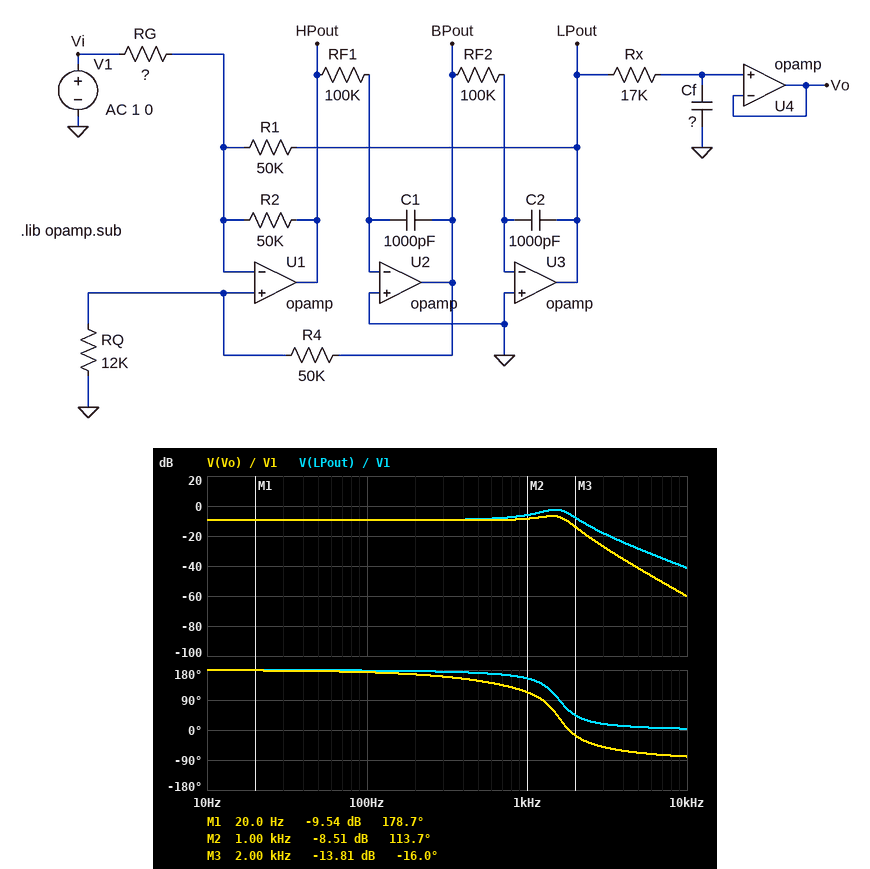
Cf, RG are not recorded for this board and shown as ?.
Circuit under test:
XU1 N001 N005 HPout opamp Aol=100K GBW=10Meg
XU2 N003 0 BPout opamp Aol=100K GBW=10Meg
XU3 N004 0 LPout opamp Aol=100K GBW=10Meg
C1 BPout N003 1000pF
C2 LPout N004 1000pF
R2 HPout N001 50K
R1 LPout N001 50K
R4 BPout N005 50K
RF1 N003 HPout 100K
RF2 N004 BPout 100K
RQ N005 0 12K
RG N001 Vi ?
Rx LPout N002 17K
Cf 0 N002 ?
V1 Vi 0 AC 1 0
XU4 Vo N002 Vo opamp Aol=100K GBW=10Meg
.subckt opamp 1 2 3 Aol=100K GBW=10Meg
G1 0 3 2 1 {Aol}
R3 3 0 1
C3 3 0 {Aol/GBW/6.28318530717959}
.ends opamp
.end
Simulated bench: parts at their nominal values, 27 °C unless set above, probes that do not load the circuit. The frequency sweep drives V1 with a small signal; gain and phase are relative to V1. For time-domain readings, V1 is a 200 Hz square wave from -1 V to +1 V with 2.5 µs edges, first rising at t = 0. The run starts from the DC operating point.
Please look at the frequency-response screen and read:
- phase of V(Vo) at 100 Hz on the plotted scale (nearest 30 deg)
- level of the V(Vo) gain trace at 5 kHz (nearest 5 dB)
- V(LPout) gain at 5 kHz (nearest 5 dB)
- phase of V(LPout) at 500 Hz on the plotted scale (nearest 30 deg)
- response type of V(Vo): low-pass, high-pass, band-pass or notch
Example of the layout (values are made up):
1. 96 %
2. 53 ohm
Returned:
1. 180 deg
2. -40 dB
3. -30 dB
4. 180 deg
5. low-pass
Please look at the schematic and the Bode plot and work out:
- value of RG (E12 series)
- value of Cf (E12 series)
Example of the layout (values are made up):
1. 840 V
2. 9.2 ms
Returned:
1. 150 kΩ
2. 8.2 nF
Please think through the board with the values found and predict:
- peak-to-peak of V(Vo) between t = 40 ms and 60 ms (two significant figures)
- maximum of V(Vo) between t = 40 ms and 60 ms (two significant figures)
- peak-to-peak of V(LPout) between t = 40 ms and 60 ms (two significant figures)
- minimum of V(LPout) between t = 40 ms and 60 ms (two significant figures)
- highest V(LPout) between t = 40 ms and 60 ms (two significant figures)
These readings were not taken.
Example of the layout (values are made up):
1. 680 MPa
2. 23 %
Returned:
1. 950 mV
2. 470 mV
3. 1.3 V
4. -660 mV
5. 660 mV
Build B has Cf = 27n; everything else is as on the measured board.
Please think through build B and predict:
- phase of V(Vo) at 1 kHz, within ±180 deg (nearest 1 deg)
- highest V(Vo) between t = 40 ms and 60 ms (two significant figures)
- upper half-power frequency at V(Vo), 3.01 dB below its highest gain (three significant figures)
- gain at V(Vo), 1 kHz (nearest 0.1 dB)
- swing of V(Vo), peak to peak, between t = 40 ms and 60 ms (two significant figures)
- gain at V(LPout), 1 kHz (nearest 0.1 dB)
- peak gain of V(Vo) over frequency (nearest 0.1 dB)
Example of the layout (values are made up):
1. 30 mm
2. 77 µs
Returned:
1. 84 deg
2. 330 mV
3. 384 Hz
4. -15.7 dB
5. 660 mV
6. -6.0 dB
7. -9.5 dB
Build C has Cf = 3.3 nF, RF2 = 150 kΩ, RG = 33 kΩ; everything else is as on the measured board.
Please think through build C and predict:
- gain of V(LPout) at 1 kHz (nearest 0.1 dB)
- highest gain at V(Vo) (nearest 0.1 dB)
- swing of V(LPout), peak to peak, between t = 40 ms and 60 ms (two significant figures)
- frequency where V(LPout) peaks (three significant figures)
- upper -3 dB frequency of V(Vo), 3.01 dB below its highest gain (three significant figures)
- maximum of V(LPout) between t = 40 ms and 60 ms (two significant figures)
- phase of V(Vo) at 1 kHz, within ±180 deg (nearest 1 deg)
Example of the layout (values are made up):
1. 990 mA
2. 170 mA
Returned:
1. 6.0 dB
2. 5.5 dB
3. 4.5 V
4. 1.05 kHz
5. 1.49 kHz
6. 2.2 V
7. 103 deg
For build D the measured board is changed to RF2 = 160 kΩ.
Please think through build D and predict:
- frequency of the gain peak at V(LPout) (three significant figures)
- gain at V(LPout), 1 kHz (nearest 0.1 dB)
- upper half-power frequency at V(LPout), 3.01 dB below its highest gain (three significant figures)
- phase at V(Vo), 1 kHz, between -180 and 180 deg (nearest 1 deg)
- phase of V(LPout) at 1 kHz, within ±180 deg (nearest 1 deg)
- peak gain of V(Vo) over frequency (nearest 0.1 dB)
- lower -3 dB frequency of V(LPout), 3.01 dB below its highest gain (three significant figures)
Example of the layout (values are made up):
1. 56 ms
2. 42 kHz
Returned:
1. 1.15 kHz
2. -4.9 dB
3. 1.48 kHz
4. 88 deg
5. 129 deg
6. -7.2 dB
7. 678 Hz
